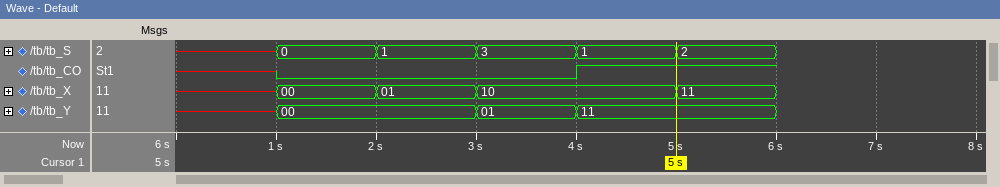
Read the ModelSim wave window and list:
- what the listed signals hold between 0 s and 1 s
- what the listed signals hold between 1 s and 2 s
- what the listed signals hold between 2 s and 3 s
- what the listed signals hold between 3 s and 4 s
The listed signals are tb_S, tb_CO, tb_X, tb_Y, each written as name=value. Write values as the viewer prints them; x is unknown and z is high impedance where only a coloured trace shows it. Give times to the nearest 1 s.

tb_S=x, tb_CO=x, tb_X=x, tb_Y=x
tb_S=0, tb_CO=0, tb_X=00, tb_Y=00
tb_S=1, tb_CO=0, tb_X=01, tb_Y=00
tb_S=3, tb_CO=0, tb_X=10, tb_Y=01
